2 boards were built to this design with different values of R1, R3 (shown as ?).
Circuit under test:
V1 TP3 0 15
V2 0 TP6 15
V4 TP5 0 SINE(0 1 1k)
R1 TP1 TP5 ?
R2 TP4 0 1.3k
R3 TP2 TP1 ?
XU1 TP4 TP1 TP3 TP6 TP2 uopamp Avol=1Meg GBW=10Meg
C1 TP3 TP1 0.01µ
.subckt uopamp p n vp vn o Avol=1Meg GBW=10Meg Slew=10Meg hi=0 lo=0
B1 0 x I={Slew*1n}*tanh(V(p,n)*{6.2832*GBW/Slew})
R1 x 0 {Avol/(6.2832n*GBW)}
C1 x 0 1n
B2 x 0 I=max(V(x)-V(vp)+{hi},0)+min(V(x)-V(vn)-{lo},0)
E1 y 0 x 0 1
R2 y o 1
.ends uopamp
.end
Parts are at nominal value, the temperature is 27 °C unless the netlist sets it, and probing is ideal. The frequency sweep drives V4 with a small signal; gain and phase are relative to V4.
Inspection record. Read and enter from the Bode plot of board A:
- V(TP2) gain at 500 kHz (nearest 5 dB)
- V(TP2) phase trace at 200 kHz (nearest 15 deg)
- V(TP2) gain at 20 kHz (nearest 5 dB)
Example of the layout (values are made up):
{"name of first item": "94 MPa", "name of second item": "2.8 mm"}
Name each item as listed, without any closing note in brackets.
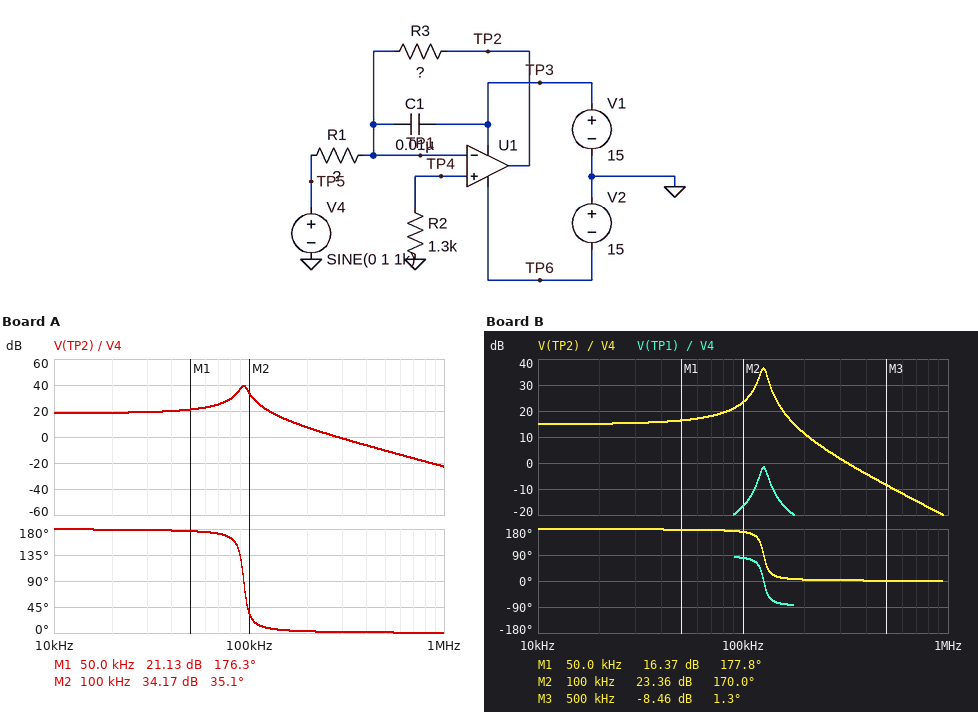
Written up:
{"V(TP2) gain at 500 kHz": "-10 dB", "V(TP2) phase trace at 200 kHz": "0 deg", "V(TP2) gain at 20 kHz": "20 dB"}
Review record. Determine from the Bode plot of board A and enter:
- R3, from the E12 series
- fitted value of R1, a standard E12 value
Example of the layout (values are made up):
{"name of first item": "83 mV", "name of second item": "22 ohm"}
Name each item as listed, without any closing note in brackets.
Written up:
{"R3, from the E12 series": "18 kΩ", "fitted value of R1, a standard E12 value": "2.2 kΩ"}
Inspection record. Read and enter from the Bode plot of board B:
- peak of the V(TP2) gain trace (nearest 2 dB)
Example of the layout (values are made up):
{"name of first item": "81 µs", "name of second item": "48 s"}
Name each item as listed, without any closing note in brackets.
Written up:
{"peak of the V(TP2) gain trace": "36 dB"}
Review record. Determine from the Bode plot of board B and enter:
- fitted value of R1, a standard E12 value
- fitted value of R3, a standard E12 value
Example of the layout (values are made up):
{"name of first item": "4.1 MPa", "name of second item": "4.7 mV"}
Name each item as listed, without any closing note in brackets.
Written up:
{"fitted value of R1, a standard E12 value": "1.8 kΩ", "fitted value of R3, a standard E12 value": "10 kΩ"}
